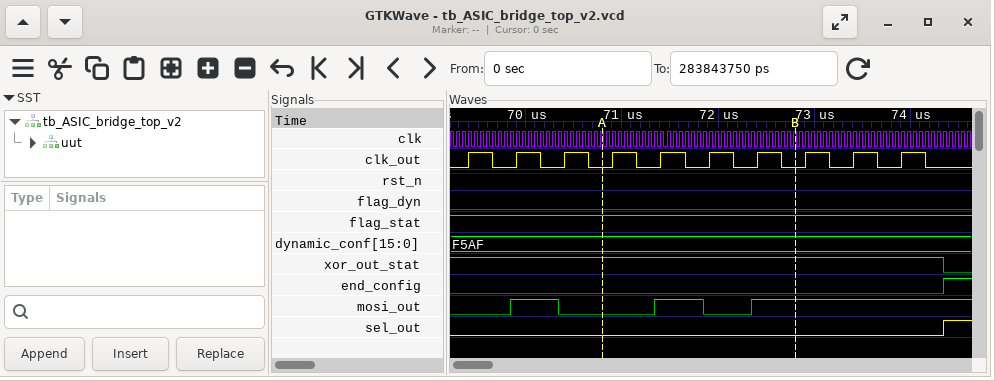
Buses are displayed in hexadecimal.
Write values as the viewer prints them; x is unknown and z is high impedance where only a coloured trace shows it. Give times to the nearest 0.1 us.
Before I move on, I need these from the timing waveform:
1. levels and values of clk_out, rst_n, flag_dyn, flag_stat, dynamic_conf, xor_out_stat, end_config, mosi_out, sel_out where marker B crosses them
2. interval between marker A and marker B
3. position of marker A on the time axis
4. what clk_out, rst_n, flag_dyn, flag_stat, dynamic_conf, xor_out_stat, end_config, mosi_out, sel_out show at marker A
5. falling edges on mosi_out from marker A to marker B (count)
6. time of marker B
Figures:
clk_out=0, rst_n=1, flag_dyn=0, flag_stat=1, dynamic_conf=F5AF, xor_out_stat=1, end_config=0, mosi_out=1, sel_out=0
2 us
70.8 us
clk_out=0, rst_n=1, flag_dyn=0, flag_stat=1, dynamic_conf=F5AF, xor_out_stat=1, end_config=0, mosi_out=0, sel_out=0
1
72.8 us
